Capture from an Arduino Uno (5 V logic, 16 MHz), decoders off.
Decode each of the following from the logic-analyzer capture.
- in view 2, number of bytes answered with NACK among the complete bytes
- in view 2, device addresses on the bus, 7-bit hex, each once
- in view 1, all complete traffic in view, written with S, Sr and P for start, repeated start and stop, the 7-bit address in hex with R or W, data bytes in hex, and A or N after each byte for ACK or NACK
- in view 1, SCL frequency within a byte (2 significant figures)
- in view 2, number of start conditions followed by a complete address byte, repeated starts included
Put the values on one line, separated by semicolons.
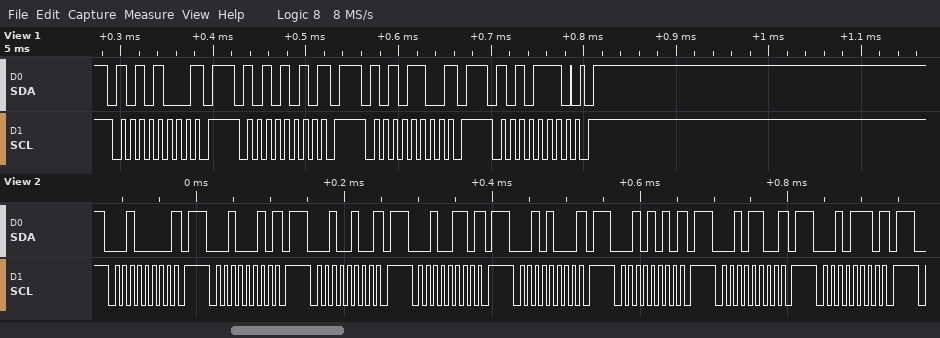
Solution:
8; 0x10 0x11 0x12 0x13 0x14 0x15 0x16 0x17; S 54W N P S 55W N P S 56W N P S 57W A P; 100 kHz; 8
